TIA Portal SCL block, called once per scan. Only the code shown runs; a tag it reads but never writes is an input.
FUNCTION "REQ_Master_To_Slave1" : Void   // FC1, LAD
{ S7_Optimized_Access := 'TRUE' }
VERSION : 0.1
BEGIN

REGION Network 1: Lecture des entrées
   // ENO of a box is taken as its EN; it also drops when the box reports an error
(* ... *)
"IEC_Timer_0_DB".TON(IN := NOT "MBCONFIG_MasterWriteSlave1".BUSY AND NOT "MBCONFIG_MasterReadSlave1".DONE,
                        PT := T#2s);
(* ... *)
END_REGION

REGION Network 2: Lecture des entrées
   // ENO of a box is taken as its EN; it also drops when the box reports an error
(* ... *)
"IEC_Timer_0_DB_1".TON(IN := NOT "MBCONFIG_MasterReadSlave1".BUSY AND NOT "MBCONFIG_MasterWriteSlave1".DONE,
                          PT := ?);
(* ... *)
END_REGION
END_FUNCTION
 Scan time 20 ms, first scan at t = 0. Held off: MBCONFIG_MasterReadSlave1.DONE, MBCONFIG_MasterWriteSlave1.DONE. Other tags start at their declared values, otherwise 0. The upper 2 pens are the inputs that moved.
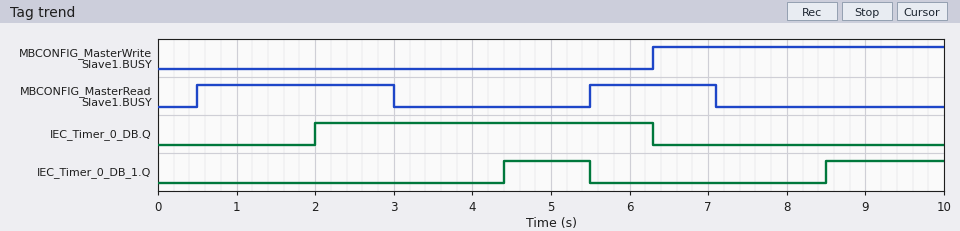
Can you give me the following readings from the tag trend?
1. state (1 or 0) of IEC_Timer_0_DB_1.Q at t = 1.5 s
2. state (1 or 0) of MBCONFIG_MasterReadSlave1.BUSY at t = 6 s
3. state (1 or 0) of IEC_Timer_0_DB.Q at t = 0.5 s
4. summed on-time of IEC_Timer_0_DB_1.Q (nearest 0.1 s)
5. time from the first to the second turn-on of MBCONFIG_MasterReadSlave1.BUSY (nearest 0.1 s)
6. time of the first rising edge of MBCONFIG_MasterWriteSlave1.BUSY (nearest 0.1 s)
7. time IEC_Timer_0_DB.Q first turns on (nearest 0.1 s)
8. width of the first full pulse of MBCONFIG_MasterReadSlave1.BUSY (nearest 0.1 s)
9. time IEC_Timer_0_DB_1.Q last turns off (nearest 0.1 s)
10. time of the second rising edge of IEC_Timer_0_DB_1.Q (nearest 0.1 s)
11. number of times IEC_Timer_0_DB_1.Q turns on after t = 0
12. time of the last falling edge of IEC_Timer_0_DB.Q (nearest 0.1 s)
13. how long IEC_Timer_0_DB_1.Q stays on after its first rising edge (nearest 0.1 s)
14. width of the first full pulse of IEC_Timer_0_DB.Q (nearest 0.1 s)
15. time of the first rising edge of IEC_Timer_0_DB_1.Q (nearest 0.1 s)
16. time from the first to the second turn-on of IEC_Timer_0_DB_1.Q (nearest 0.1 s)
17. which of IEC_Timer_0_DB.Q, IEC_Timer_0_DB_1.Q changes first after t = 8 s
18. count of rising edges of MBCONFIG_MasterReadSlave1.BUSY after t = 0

0
1
0
2.6 s
5.0 s
6.3 s
2.0 s
2.5 s
5.5 s
8.5 s
2
6.3 s
1.1 s
4.3 s
4.4 s
4.1 s
IEC_Timer_0_DB_1.Q
2
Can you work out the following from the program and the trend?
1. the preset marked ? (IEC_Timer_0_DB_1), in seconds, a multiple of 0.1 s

1.4 s
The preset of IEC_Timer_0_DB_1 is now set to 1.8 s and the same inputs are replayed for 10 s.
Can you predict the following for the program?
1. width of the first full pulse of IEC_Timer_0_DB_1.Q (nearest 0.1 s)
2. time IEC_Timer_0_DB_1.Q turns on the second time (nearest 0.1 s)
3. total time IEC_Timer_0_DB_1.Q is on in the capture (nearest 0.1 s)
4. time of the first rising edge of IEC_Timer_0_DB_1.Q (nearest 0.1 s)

0.7 s
8.9 s
1.8 s
4.8 s
